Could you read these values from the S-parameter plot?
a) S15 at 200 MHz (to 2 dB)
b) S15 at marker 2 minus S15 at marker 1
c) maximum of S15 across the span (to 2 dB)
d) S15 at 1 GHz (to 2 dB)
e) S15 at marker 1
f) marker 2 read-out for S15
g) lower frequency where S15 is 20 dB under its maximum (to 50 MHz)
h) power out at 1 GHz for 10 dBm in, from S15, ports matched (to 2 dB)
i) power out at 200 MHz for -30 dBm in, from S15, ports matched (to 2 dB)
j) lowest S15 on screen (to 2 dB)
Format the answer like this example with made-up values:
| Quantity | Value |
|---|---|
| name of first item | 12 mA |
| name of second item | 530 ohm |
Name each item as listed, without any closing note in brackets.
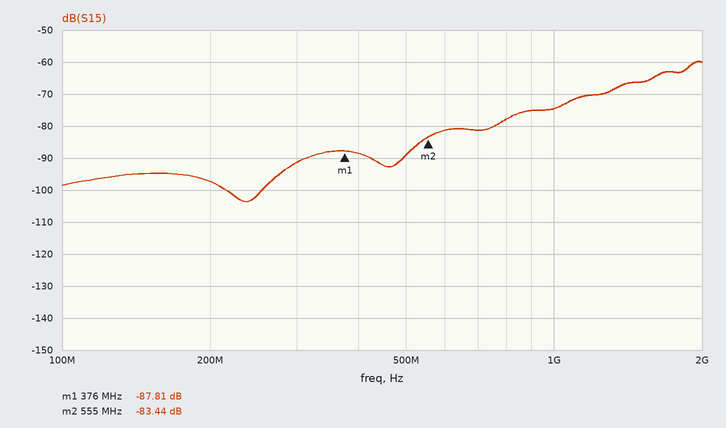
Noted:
| Quantity | Value |
|---|---|
| S15 at 200 MHz | -98 dB |
| S15 at marker 2 minus S15 at marker 1 | 4.37 dB |
| maximum of S15 across the span | -60 dB |
| S15 at 1 GHz | -74 dB |
| S15 at marker 1 | -87.81 dB |
| marker 2 read-out for S15 | -83.44 dB |
| lower frequency where S15 is 20 dB under its maximum | 750 MHz |
| power out at 1 GHz for 10 dBm in, from S15, ports matched | -64 dBm |
| power out at 200 MHz for -30 dBm in, from S15, ports matched | -128 dBm |
| lowest S15 on screen | -104 dB |
